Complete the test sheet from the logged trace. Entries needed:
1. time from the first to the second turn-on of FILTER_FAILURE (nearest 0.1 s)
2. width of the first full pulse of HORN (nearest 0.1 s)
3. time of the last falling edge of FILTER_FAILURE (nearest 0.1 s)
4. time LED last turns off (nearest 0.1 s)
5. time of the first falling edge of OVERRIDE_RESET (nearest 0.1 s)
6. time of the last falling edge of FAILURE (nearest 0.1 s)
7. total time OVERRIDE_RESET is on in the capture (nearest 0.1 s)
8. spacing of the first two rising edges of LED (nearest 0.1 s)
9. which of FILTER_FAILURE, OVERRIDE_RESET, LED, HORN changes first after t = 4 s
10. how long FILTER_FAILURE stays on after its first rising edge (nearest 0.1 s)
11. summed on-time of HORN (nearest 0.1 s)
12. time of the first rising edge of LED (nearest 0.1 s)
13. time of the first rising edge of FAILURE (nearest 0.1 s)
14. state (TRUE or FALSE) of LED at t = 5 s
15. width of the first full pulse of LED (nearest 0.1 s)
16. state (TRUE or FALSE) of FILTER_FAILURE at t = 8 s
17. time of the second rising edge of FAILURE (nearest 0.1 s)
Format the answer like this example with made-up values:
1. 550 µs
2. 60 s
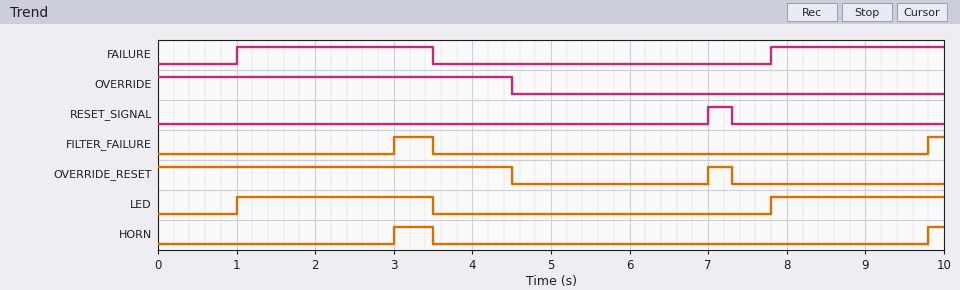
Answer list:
1. 6.8 s
2. 0.5 s
3. 3.5 s
4. 3.5 s
5. 4.5 s
6. 3.5 s
7. 4.8 s
8. 6.8 s
9. OVERRIDE_RESET
10. 0.5 s
11. 0.7 s
12. 1.0 s
13. 1.0 s
14. FALSE
15. 2.5 s
16. FALSE
17. 7.8 s
